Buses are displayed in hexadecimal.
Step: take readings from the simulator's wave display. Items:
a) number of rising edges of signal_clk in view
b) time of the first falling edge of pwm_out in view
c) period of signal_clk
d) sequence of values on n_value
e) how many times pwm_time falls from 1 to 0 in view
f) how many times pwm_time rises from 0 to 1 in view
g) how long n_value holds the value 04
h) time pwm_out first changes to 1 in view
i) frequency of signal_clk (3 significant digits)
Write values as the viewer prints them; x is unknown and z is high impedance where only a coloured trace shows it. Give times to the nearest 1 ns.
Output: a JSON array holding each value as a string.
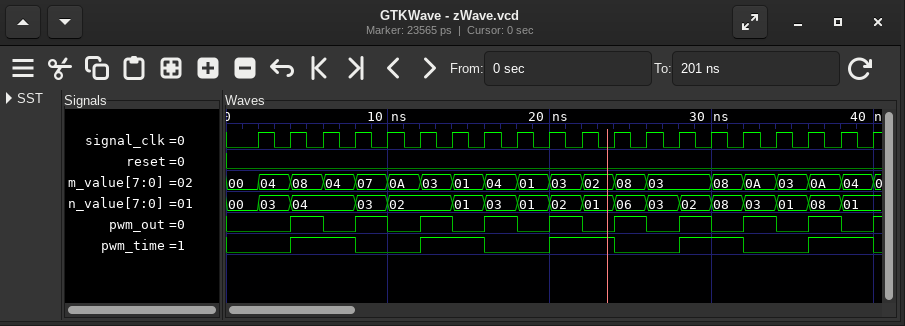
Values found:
["20", "6 ns", "2 ns", "00, 03, 04, 03, 02, 01, 03, 01, 02, 01, 06, 03, 02, 08, 03, 01, 08, 01", "5", "5", "4 ns", "4 ns", "500 MHz"]
